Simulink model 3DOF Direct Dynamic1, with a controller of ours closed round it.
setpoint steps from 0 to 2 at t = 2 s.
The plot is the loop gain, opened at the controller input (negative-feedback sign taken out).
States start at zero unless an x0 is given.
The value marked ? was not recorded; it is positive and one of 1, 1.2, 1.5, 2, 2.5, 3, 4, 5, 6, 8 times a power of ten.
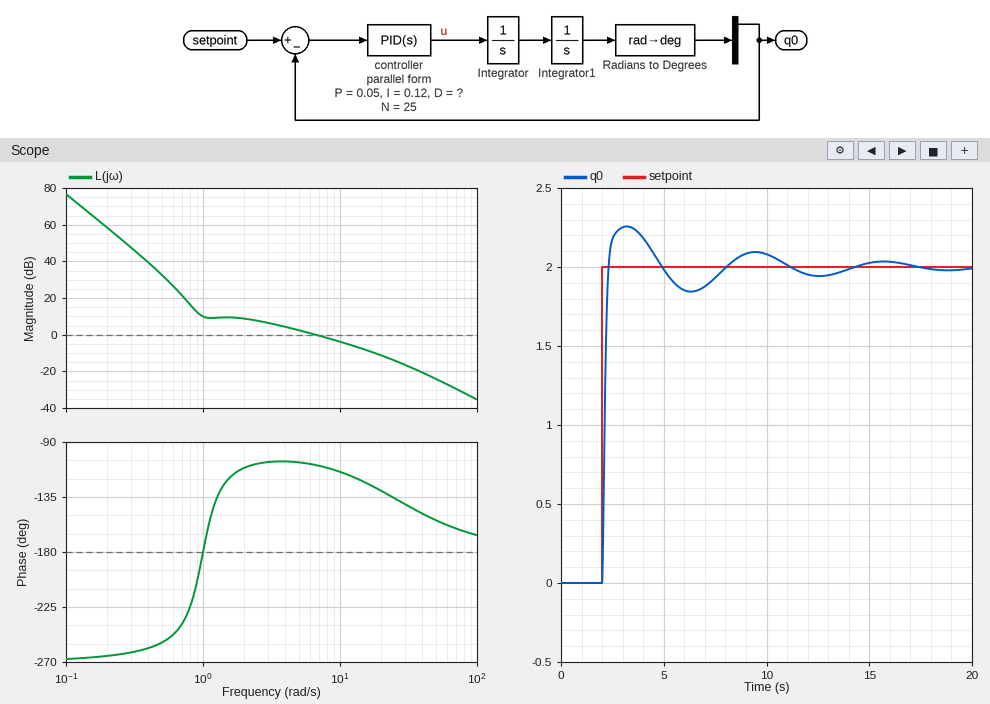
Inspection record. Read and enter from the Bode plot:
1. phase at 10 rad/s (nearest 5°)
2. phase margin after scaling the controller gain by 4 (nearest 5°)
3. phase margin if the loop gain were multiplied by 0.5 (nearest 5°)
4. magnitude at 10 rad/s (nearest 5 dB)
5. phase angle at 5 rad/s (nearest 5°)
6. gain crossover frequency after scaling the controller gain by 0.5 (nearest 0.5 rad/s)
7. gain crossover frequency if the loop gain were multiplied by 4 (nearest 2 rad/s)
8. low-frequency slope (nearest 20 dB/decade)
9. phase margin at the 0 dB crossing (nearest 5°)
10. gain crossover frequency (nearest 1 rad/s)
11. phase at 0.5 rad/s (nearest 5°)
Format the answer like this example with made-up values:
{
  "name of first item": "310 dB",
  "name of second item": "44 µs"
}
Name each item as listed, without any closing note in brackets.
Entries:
{
  "phase at 10 rad/s": "-115°",
  "phase margin after scaling the controller gain by 4": "50°",
  "phase margin if the loop gain were multiplied by 0.5": "75°",
  "magnitude at 10 rad/s": "-5 dB",
  "phase angle at 5 rad/s": "-105°",
  "gain crossover frequency after scaling the controller gain by 0.5": "3.0 rad/s",
  "gain crossover frequency if the loop gain were multiplied by 4": "22 rad/s",
  "low-frequency slope": "-60 dB/decade",
  "phase margin at the 0 dB crossing": "70°",
  "gain crossover frequency": "7 rad/s",
  "phase at 0.5 rad/s": "-255°"
}
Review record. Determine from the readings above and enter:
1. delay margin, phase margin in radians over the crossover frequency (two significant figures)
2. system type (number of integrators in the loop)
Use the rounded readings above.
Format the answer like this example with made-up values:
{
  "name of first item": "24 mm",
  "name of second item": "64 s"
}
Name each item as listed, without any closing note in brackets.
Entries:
{
  "delay margin, phase margin in radians over the crossover frequency": "0.17 s",
  "system type": "3"
}
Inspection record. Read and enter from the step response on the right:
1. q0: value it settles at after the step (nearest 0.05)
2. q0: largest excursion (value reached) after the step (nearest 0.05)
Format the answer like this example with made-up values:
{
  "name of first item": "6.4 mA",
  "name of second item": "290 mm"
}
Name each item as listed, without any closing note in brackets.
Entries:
{
  "q0: value it settles at after the step": "2.00",
  "q0: largest excursion (value reached) after the step": "2.25"
}
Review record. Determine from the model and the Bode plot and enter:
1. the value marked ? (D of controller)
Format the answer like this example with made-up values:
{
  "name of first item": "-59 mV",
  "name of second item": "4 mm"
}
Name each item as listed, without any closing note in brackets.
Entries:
{
  "the value marked ?": "0.12"
}
